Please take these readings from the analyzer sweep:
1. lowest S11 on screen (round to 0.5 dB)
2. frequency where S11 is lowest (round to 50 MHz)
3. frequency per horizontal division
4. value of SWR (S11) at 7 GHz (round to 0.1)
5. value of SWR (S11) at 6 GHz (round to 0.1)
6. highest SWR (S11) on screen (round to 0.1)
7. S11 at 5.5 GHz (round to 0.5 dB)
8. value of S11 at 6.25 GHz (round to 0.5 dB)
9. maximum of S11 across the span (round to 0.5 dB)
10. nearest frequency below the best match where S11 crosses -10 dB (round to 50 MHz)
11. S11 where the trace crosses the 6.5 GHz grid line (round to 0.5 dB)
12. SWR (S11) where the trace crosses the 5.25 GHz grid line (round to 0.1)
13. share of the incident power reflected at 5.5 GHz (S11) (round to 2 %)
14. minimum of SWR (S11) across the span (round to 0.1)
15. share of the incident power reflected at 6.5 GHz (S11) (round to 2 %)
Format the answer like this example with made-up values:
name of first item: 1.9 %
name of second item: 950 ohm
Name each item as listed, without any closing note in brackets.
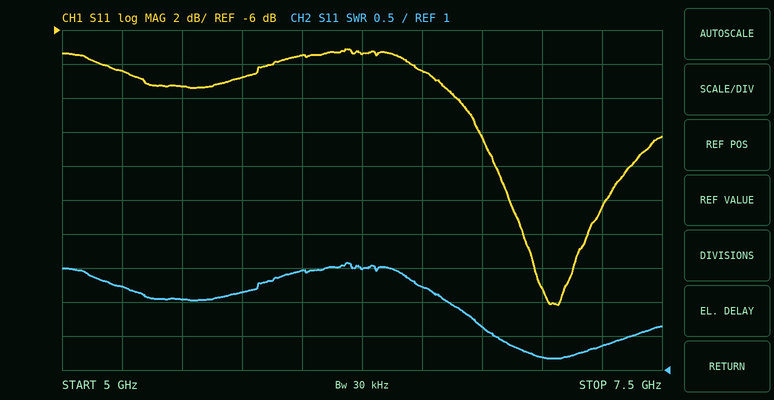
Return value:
lowest S11 on screen: -22.0 dB
frequency where S11 is lowest: 7.05 GHz
frequency per horizontal division: 250 MHz
value of SWR (S11) at 7 GHz: 1.2
value of SWR (S11) at 6 GHz: 2.5
highest SWR (S11) on screen: 2.6
S11 at 5.5 GHz: -9.5 dB
value of S11 at 6.25 GHz: -7.5 dB
maximum of S11 across the span: -7.0 dB
nearest frequency below the best match where S11 crosses -10 dB: 6.65 GHz
S11 where the trace crosses the 6.5 GHz grid line: -8.5 dB
SWR (S11) where the trace crosses the 5.25 GHz grid line: 2.2
share of the incident power reflected at 5.5 GHz (S11): 12 %
minimum of SWR (S11) across the span: 1.2
share of the incident power reflected at 6.5 GHz (S11): 14 %
